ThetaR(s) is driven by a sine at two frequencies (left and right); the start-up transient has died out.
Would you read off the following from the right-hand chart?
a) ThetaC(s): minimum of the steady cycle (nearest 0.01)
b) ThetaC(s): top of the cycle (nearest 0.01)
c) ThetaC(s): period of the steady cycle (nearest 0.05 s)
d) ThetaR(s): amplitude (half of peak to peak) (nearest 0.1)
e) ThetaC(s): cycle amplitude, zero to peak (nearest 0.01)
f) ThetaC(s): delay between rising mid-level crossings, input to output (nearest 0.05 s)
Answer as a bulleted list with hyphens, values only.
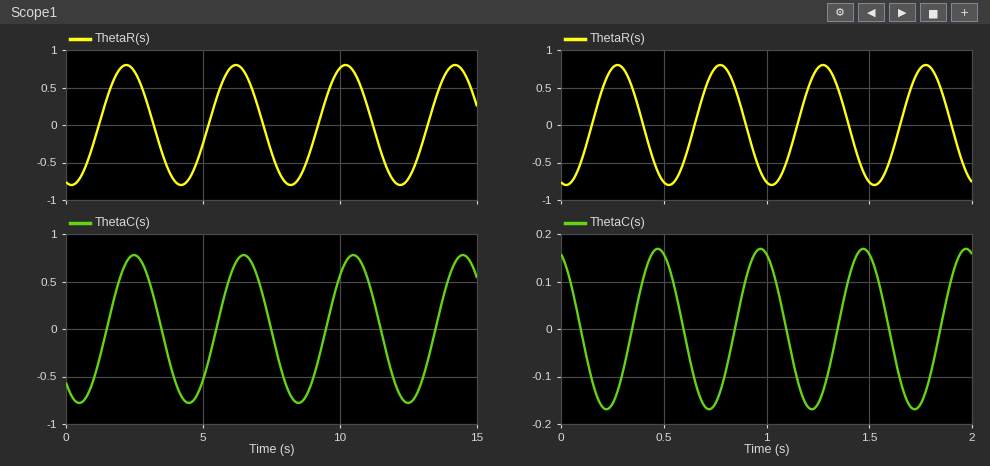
- -0.17
- 0.17
- 0.50 s
- 0.8
- 0.17
- 0.20 s
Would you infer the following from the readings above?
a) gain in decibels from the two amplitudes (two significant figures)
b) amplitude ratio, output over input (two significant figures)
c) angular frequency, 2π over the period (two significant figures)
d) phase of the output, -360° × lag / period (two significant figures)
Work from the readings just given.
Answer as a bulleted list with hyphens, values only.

- -13 dB
- 0.21
- 13 rad/s
- -140°
